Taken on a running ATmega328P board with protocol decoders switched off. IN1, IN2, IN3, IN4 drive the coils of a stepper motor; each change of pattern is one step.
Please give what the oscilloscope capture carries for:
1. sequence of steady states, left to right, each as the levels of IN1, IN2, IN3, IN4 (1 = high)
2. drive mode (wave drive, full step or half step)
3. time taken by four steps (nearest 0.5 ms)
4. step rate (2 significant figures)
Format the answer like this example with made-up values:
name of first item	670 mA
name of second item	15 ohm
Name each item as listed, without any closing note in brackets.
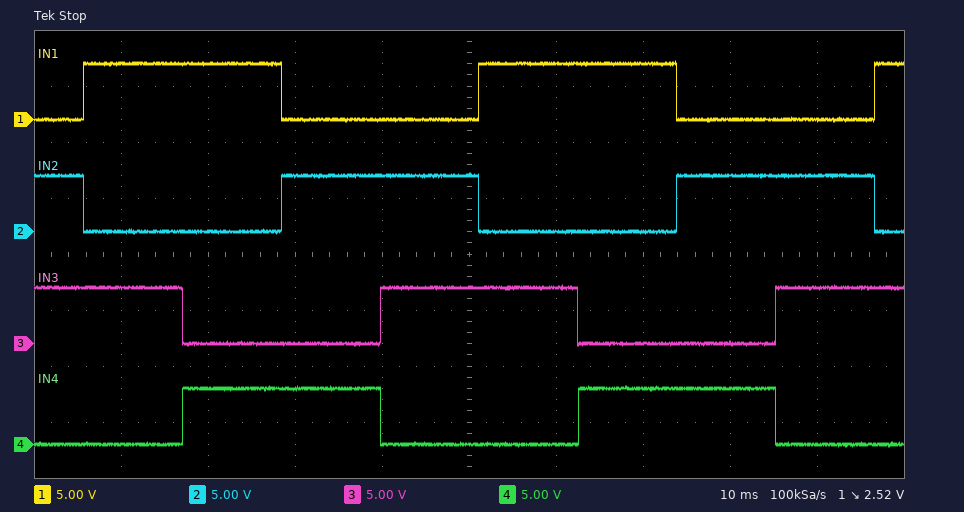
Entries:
sequence of steady states, left to right, each as the levels of IN1, IN2, IN3, IN4	0110 1010 1001 0101 0110 1010 1001 0101 0110 1010
drive mode	full step
time taken by four steps	45.5 ms
step rate	88 steps/s
